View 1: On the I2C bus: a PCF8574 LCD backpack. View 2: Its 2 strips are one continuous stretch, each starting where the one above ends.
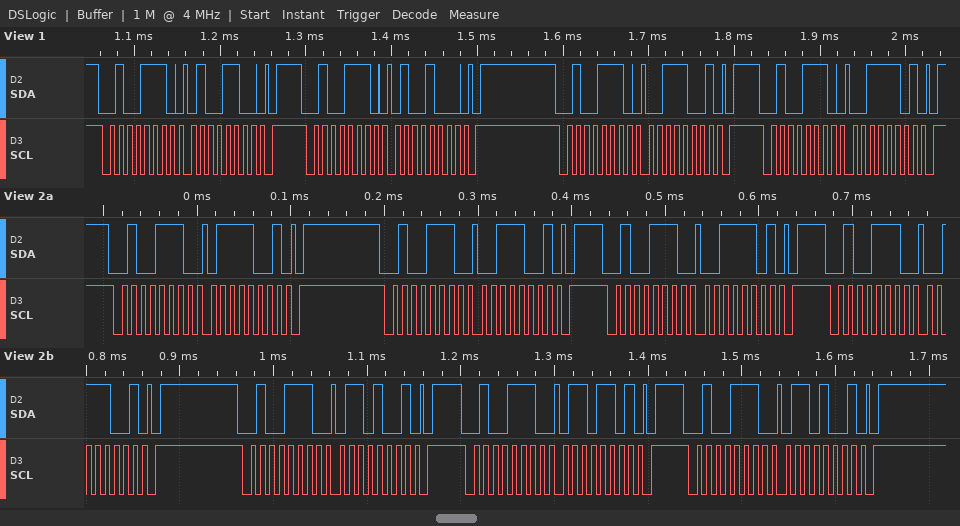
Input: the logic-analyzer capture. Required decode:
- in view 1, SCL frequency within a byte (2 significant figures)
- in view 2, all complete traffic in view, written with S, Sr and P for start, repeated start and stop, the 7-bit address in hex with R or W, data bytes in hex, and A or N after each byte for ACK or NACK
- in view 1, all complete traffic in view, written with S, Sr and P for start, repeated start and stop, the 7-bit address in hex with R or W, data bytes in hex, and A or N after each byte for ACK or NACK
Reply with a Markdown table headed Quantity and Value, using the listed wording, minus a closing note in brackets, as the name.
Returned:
| Quantity | Value |
|---|---|
| in view 1, SCL frequency within a byte | 100 kHz |
| in view 2, all complete traffic in view, written with S, Sr and P for start, repeated start and stop, the 7-bit address in hex with R or W, data bytes in hex, and A or N after each byte for ACK or NACK | S 27W A 79 A P S 27W A 39 A P S 27W A 3D A P S 27W A 39 A P S 27W A 69 A P S 27W A 6D A P S 27W A 69 A P |
| in view 1, all complete traffic in view, written with S, Sr and P for start, repeated start and stop, the 7-bit address in hex with R or W, data bytes in hex, and A or N after each byte for ACK or NACK | S 27W A 4C A P S 27W A 48 A P S 27W A 39 A P S 27W A 3D A P |
